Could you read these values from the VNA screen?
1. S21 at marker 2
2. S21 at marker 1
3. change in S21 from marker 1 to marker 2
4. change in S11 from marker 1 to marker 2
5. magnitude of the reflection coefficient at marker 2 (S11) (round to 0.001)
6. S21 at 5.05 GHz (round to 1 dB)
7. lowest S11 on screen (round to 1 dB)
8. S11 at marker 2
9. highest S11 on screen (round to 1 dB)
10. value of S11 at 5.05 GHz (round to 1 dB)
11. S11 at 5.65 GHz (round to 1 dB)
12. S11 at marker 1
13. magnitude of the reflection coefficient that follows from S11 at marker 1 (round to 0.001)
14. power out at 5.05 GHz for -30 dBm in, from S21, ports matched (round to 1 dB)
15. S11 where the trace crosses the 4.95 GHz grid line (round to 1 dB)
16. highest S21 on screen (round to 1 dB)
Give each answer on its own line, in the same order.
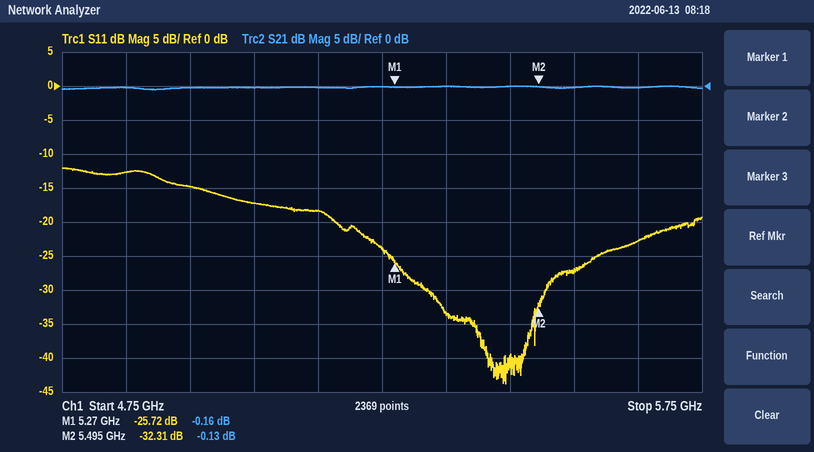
-0.13 dB
-0.16 dB
0.03 dB
-6.59 dB
0.024
0 dB
-44 dB
-32.31 dB
-12 dB
-17 dB
-23 dB
-25.72 dB
0.052
-30 dBm
-15 dB
0 dB
